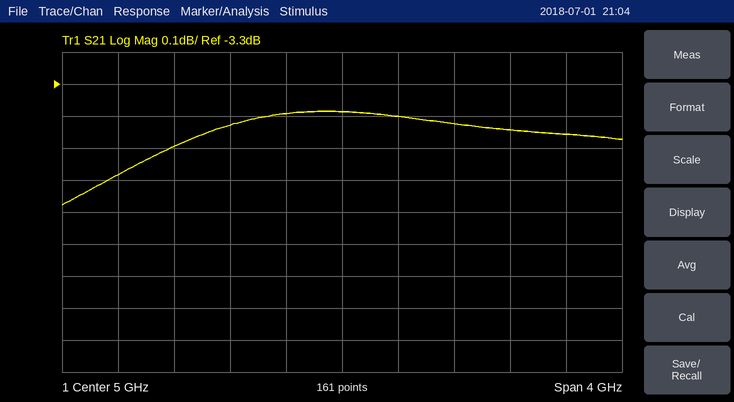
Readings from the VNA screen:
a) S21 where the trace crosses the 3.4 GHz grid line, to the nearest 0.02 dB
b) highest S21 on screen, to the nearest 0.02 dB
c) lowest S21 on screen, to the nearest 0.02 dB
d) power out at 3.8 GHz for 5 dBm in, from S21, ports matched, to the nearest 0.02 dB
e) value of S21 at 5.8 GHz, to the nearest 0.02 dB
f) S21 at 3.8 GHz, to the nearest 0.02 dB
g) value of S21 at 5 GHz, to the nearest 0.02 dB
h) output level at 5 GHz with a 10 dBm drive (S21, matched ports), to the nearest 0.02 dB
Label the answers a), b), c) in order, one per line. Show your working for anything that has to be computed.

a) -3.58 dB
b) -3.38 dB
c) -3.68 dB
d) 5 dBm + (-3.50 dB) = 1.50 dBm
e) -3.42 dB
f) -3.50 dB
g) -3.38 dB
h) 10 dBm + (-3.38 dB) = 6.62 dBm
